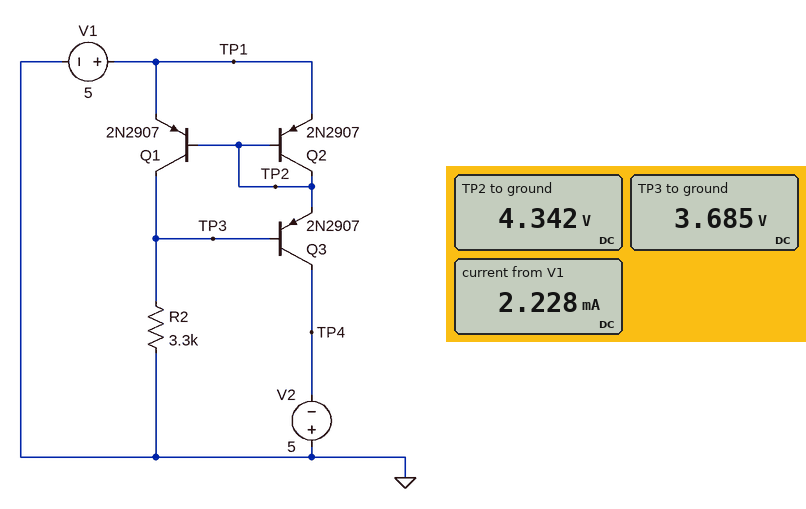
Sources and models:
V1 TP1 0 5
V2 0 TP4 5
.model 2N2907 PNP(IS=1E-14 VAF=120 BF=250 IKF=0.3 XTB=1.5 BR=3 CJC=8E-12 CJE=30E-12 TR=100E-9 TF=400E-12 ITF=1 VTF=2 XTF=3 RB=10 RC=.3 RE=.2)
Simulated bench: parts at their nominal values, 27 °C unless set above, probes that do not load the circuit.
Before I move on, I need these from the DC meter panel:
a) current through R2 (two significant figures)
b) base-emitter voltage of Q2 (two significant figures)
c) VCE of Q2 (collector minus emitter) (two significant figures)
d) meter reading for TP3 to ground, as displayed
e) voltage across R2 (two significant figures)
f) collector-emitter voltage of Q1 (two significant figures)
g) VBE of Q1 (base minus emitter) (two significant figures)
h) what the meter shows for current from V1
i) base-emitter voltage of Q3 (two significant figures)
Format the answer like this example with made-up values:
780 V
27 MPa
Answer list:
1.1 mA
-660 mV
-660 mV
3.685 V
3.7 V
-1.3 V
-660 mV
2.228 mA
-660 mV
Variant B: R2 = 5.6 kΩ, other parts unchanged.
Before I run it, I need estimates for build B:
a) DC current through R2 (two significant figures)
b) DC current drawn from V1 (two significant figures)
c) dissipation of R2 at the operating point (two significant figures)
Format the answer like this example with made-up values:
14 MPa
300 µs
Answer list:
660 µA
1.3 mA
2.5 mW
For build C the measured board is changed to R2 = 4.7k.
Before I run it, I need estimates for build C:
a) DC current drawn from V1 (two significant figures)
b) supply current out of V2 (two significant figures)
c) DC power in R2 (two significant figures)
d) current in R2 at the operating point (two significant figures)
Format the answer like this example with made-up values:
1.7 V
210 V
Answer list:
1.6 mA
780 µA
2.9 mW
790 µA
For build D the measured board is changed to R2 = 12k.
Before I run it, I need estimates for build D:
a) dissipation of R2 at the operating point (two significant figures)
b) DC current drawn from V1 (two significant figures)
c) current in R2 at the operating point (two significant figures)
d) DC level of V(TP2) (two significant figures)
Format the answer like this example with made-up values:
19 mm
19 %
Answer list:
1.2 mW
620 µA
310 µA
4.4 V
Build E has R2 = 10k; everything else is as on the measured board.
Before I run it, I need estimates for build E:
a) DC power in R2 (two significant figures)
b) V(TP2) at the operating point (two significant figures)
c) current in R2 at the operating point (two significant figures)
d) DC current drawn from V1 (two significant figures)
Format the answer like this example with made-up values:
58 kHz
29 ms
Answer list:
1.4 mW
4.4 V
370 µA
750 µA
